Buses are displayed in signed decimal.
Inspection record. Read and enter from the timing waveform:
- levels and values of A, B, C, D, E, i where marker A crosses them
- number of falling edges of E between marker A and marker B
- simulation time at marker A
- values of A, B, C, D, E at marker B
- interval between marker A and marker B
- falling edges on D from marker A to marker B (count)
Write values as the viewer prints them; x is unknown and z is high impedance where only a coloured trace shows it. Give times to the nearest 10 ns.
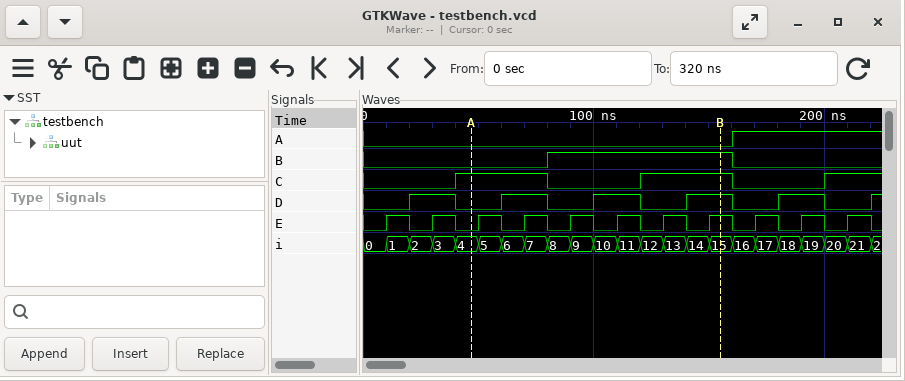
A=0, B=0, C=1, D=0, E=0, i=4
5
50 ns
A=0, B=1, C=1, D=1, E=1
110 ns
2
